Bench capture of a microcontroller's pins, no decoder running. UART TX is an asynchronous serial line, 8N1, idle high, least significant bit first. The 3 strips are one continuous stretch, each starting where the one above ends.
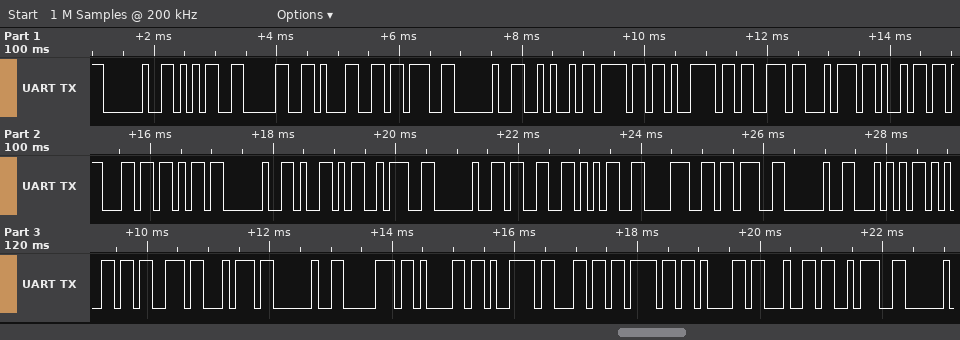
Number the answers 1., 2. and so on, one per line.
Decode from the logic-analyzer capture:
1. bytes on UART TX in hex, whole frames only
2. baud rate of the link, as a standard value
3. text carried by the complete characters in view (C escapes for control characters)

1. 20 35 30 31 3B 20 4A 6F 79 73 74 69 63 6B 20 59 3A 20 33 35 38 3B 20 54 65 73 74 20 70 61 79 6C 6F 61 64 3A
2. 9600 baud
3. " 501; Joystick Y: 358; Test payload:"
